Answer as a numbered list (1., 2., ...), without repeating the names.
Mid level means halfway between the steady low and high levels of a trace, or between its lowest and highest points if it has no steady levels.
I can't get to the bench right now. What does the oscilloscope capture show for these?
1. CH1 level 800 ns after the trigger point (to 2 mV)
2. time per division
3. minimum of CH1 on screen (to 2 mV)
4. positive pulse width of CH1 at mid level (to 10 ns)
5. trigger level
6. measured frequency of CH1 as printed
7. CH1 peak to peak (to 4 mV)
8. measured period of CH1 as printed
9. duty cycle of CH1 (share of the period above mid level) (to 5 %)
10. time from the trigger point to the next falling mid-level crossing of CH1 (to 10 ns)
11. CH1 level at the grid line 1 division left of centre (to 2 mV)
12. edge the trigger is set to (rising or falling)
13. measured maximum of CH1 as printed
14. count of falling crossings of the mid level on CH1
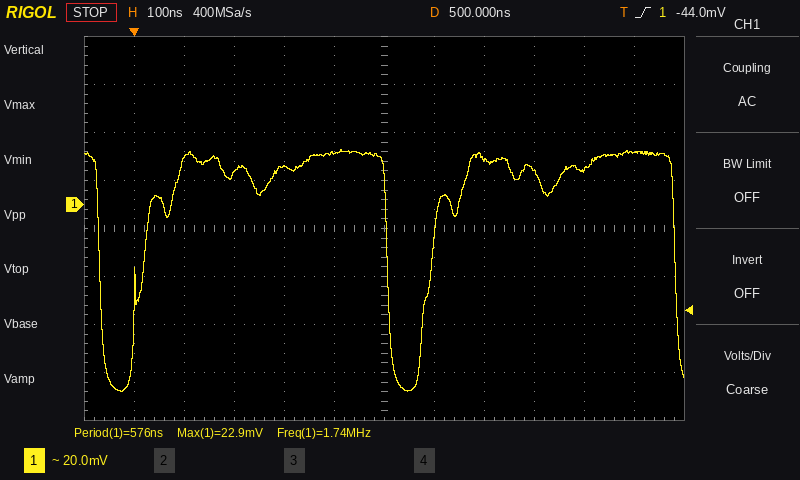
1. 14 mV
2. 100 ns
3. -78 mV
4. 490 ns
5. -44.0 mV
6. 1.74 MHz
7. 100 mV
8. 576 ns
9. 85 %
10. 510 ns
11. 22 mV
12. rising
13. 22.9 mV
14. 3
